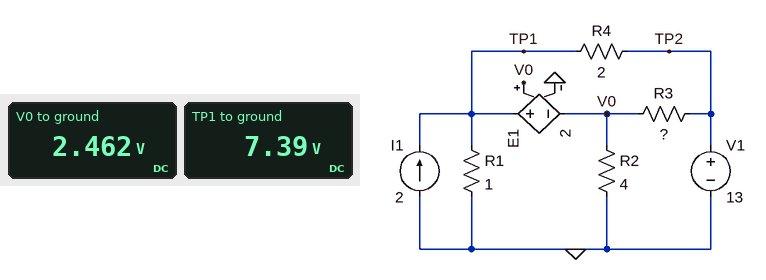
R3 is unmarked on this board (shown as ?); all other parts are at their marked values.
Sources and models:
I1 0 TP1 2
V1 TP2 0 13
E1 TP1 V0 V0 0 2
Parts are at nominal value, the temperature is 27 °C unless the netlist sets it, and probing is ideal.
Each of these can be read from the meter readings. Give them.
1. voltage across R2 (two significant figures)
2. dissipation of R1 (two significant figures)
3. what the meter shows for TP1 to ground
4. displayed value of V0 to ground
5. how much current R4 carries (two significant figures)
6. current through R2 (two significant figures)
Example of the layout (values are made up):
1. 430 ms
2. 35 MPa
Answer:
1. 2.5 V
2. 55 W
3. 7.39 V
4. 2.462 V
5. 2.8 A
6. 620 mA
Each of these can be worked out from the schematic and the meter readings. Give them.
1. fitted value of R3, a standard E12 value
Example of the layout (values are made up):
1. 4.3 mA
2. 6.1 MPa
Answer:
1. 3.3 Ω
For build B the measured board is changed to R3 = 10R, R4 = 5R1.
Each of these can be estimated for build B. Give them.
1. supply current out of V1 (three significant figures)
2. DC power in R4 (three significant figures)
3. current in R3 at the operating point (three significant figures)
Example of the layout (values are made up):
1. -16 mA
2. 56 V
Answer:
1. 2.83 A
2. 14.3 W
3. 1.15 A
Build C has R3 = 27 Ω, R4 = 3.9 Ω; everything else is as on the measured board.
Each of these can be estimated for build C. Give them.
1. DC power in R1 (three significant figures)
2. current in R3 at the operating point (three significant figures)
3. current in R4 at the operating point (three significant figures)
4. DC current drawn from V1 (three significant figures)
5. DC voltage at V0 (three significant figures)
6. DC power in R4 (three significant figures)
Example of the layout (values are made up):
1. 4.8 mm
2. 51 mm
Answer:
1. 18.5 W
2. 428 mA
3. 2.23 A
4. 2.66 A
5. 1.43 V
6. 19.4 W
